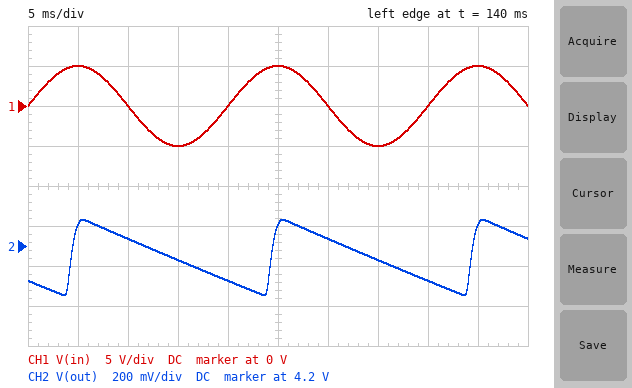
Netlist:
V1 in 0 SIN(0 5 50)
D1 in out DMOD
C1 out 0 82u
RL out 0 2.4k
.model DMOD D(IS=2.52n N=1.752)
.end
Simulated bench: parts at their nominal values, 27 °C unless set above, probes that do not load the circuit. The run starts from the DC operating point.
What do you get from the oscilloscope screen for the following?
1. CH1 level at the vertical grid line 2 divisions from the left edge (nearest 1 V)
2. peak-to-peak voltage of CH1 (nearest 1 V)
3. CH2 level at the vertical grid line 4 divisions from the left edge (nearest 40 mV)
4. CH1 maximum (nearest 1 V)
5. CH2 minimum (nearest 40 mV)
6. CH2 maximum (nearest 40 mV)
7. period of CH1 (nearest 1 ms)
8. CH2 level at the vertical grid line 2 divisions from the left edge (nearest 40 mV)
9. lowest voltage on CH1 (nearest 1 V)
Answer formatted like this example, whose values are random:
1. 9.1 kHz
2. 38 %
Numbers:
1. 0 V
2. 10 V
3. 4.04 V
4. 5 V
5. 3.96 V
6. 4.32 V
7. 20 ms
8. 4.24 V
9. -5 V
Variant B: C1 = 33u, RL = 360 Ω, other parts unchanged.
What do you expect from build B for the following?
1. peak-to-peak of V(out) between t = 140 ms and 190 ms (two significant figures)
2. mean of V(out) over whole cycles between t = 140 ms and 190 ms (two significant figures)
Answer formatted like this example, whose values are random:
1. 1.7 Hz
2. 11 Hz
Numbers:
1. 3.1 V
2. 2.6 V
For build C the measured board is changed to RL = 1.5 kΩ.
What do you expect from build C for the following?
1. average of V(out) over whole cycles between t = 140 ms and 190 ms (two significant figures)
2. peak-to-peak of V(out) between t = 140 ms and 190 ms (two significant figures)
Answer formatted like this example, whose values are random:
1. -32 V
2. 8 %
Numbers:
1. 4.0 V
2. 580 mV
